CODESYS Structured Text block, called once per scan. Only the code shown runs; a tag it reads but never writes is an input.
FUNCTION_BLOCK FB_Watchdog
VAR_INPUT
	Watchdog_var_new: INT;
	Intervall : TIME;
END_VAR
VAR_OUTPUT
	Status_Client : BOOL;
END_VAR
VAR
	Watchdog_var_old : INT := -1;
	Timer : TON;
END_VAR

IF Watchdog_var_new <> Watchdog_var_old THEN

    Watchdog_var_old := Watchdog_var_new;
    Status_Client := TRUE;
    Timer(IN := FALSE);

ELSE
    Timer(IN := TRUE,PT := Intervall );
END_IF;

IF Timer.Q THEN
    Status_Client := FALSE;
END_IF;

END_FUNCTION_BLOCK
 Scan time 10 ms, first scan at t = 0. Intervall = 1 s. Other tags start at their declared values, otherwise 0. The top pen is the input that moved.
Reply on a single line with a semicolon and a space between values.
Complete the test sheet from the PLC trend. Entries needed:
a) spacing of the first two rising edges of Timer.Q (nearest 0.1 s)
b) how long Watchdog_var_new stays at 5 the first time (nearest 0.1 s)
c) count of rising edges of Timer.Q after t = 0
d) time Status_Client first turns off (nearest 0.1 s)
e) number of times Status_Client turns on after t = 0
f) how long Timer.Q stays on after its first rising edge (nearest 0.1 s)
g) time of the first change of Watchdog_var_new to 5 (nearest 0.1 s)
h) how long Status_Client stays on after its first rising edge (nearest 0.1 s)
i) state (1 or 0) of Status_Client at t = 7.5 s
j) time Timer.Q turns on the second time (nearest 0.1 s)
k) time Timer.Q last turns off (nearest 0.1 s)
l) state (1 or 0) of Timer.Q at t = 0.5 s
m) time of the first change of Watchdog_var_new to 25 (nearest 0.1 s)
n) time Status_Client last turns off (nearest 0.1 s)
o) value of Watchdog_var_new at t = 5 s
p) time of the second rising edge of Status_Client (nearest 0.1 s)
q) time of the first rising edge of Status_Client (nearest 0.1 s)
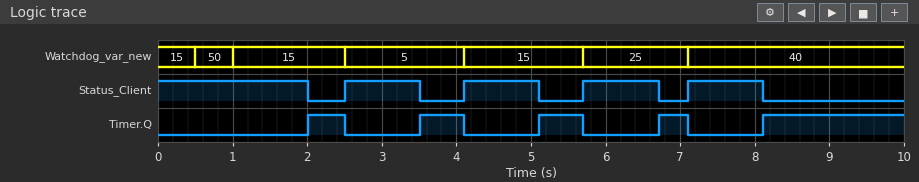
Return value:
1.5 s; 1.6 s; 5; 2.0 s; 4; 0.5 s; 2.5 s; 1.0 s; 1; 3.5 s; 7.1 s; 0; 5.7 s; 8.1 s; 15; 4.1 s; 2.5 s
